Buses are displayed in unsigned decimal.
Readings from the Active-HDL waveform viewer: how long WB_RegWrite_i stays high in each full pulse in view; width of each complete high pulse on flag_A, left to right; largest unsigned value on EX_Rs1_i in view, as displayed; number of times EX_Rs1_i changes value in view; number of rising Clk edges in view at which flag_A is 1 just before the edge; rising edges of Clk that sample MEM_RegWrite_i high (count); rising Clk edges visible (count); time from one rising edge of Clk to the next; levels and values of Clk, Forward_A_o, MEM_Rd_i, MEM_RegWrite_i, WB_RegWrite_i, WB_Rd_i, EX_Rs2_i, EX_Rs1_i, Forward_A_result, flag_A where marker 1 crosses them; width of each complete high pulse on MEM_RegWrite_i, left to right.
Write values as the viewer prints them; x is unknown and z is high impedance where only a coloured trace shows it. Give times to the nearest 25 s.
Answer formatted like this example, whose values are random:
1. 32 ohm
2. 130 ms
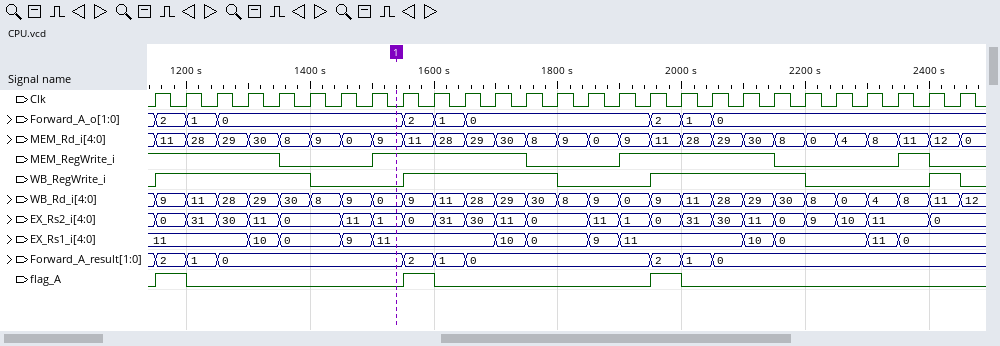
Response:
1. 250 s, 250 s, 250 s, 50 s
2. 50 s, 50 s, 50 s
3. 11
4. 12
5. 3
6. 16
7. 27
8. 50 s
9. Clk=0, Forward_A_o=0, MEM_Rd_i=9, MEM_RegWrite_i=1, WB_RegWrite_i=0, WB_Rd_i=0, EX_Rs2_i=1, EX_Rs1_i=11, Forward_A_result=0, flag_A=0
10. 250 s, 250 s, 50 s
